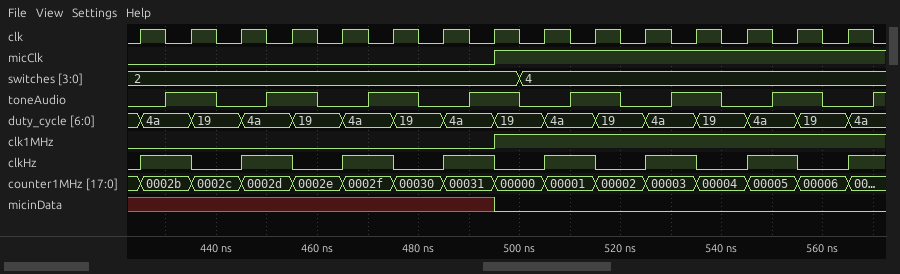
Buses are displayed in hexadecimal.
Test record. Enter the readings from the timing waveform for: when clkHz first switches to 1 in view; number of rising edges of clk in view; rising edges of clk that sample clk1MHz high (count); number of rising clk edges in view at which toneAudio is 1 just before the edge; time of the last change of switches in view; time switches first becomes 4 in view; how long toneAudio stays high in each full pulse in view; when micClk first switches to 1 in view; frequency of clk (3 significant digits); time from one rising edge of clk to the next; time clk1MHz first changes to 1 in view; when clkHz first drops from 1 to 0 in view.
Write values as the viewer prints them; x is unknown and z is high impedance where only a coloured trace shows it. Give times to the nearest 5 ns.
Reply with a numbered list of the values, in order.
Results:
1. 425 ns
2. 15
3. 7
4. 7
5. 500 ns
6. 500 ns
7. 10 ns, 10 ns, 10 ns, 10 ns, 10 ns, 10 ns, 10 ns
8. 495 ns
9. 100 MHz
10. 10 ns
11. 495 ns
12. 435 ns
